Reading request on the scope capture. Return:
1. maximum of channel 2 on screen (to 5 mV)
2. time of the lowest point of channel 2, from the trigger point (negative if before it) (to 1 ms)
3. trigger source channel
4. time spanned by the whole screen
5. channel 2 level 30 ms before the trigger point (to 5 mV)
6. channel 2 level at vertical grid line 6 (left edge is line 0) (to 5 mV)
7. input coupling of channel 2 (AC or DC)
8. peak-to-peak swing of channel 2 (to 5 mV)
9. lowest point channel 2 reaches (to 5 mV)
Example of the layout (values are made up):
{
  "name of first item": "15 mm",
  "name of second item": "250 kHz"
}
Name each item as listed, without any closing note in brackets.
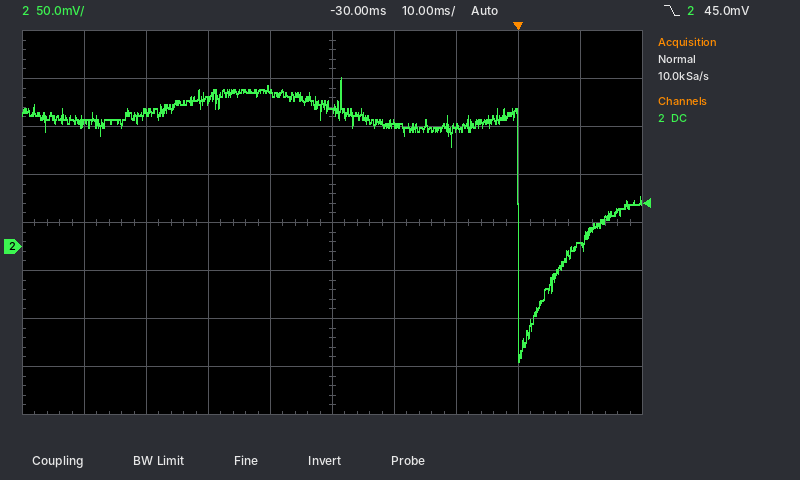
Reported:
{
  "maximum of channel 2 on screen": "175 mV",
  "time of the lowest point of channel 2, from the trigger point (negative if before it)": "0 ms",
  "trigger source channel": "channel 2",
  "time spanned by the whole screen": "100 ms",
  "channel 2 level 30 ms before the trigger point": "145 mV",
  "channel 2 level at vertical grid line 6 (left edge is line 0)": "130 mV",
  "input coupling of channel 2": "DC",
  "peak-to-peak swing of channel 2": "295 mV",
  "lowest point channel 2 reaches": "-120 mV"
}
